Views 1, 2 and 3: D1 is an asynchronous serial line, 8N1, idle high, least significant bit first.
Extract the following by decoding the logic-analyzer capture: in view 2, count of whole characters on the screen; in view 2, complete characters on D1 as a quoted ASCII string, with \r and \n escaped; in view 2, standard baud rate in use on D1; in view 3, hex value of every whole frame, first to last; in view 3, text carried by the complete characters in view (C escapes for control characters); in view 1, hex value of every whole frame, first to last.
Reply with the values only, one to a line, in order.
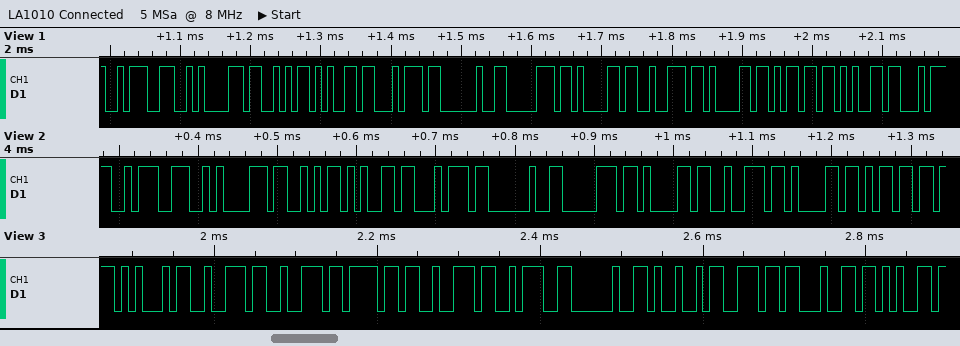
11
":\nSet param"
115200 baud
45 72 72 6F 72 3A 20 49 6E 64 65
"Error: Inde"
3A 0A 53 65 74 20 70 61 72 61 6D 65
